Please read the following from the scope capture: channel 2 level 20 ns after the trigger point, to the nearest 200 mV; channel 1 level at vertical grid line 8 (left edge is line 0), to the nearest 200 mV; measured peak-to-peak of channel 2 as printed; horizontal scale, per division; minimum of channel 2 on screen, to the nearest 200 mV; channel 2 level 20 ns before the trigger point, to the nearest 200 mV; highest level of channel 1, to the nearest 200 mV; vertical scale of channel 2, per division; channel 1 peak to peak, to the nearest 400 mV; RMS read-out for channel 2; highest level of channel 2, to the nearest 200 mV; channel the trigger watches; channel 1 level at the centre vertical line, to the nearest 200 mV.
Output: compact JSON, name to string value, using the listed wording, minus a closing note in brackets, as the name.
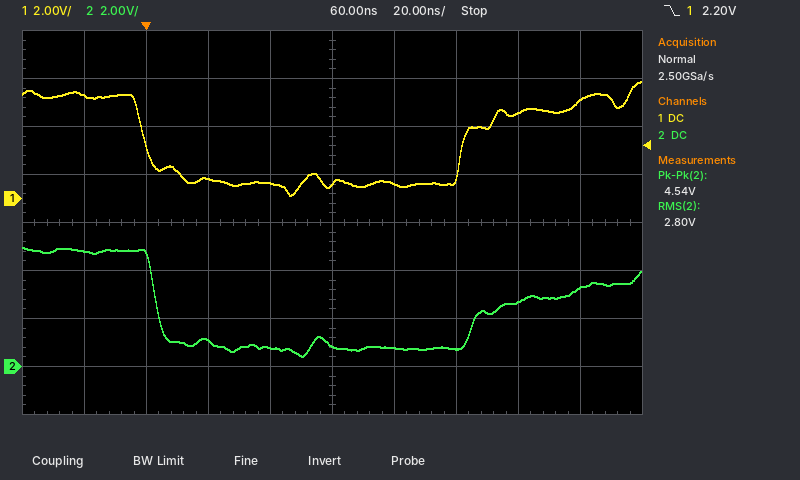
{"channel 2 level 20 ns after the trigger point, to the nearest 200 mV": "1.0 V", "channel 1 level at vertical grid line 8 (left edge is line 0), to the nearest 200 mV": "3.6 V", "measured peak-to-peak of channel 2 as printed": "4.54 V", "horizontal scale, per division": "20 ns", "minimum of channel 2 on screen, to the nearest 200 mV": "400 mV", "channel 2 level 20 ns before the trigger point, to the nearest 200 mV": "4.8 V", "highest level of channel 1, to the nearest 200 mV": "4.8 V", "vertical scale of channel 2, per division": "2 V", "channel 1 peak to peak, to the nearest 400 mV": "4.8 V", "RMS read-out for channel 2": "2.80 V", "highest level of channel 2, to the nearest 200 mV": "5.0 V", "channel the trigger watches": "channel 1", "channel 1 level at the centre vertical line, to the nearest 200 mV": "600 mV"}
